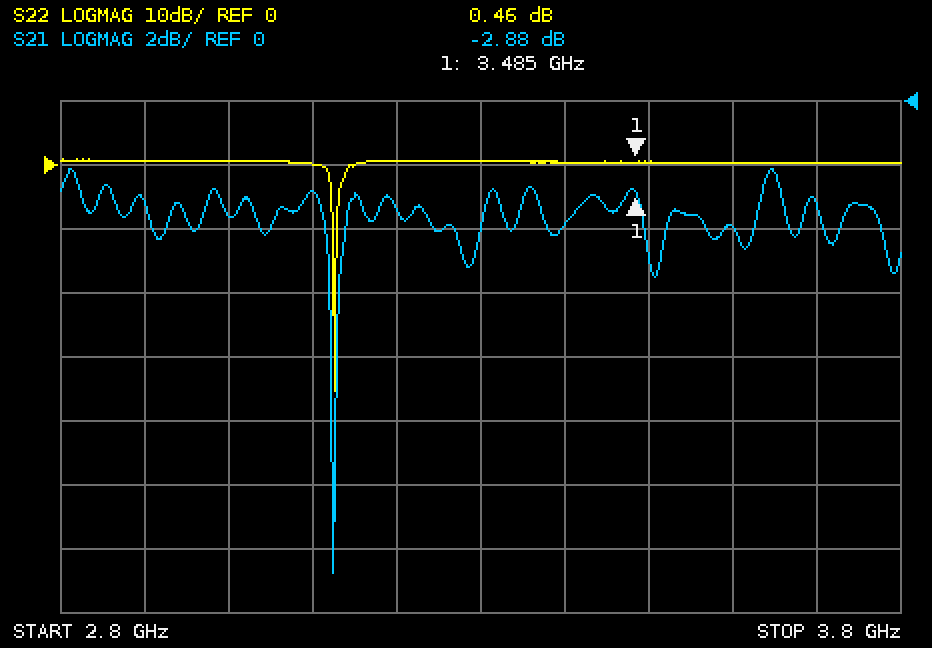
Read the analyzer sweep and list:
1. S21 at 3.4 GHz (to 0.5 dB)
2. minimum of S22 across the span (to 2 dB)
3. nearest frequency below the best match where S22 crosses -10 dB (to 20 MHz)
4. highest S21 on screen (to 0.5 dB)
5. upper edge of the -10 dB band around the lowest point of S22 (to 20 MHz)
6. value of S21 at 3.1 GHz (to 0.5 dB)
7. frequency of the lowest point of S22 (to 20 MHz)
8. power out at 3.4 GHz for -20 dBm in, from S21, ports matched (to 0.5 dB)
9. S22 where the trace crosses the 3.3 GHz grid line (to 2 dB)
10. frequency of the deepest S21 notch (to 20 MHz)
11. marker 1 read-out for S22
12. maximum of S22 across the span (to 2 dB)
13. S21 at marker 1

-4.0 dB
-36 dB
3.12 GHz
-2.0 dB
3.12 GHz
-3.0 dB
3.12 GHz
-24.0 dBm
0 dB
3.12 GHz
0.46 dB
0 dB
-2.88 dB
